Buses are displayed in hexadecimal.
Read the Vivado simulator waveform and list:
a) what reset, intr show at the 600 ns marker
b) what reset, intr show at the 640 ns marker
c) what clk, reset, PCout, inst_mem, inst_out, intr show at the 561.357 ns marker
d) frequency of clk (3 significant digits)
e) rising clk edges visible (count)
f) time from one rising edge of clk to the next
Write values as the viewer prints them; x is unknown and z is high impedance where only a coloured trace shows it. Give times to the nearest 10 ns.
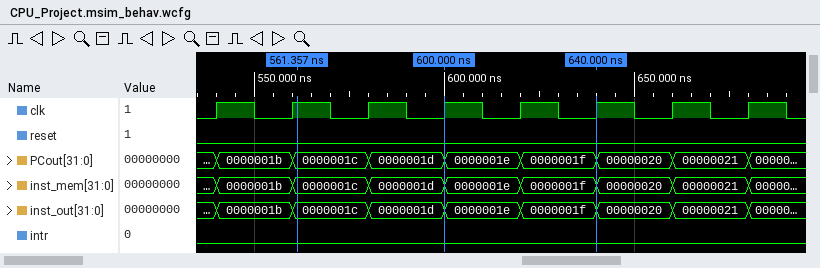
reset=0, intr=0
reset=0, intr=0
clk=1, reset=0, PCout=0000001c, inst_mem=0000001c, inst_out=0000001c, intr=0
50.0 MHz
8
20 ns
